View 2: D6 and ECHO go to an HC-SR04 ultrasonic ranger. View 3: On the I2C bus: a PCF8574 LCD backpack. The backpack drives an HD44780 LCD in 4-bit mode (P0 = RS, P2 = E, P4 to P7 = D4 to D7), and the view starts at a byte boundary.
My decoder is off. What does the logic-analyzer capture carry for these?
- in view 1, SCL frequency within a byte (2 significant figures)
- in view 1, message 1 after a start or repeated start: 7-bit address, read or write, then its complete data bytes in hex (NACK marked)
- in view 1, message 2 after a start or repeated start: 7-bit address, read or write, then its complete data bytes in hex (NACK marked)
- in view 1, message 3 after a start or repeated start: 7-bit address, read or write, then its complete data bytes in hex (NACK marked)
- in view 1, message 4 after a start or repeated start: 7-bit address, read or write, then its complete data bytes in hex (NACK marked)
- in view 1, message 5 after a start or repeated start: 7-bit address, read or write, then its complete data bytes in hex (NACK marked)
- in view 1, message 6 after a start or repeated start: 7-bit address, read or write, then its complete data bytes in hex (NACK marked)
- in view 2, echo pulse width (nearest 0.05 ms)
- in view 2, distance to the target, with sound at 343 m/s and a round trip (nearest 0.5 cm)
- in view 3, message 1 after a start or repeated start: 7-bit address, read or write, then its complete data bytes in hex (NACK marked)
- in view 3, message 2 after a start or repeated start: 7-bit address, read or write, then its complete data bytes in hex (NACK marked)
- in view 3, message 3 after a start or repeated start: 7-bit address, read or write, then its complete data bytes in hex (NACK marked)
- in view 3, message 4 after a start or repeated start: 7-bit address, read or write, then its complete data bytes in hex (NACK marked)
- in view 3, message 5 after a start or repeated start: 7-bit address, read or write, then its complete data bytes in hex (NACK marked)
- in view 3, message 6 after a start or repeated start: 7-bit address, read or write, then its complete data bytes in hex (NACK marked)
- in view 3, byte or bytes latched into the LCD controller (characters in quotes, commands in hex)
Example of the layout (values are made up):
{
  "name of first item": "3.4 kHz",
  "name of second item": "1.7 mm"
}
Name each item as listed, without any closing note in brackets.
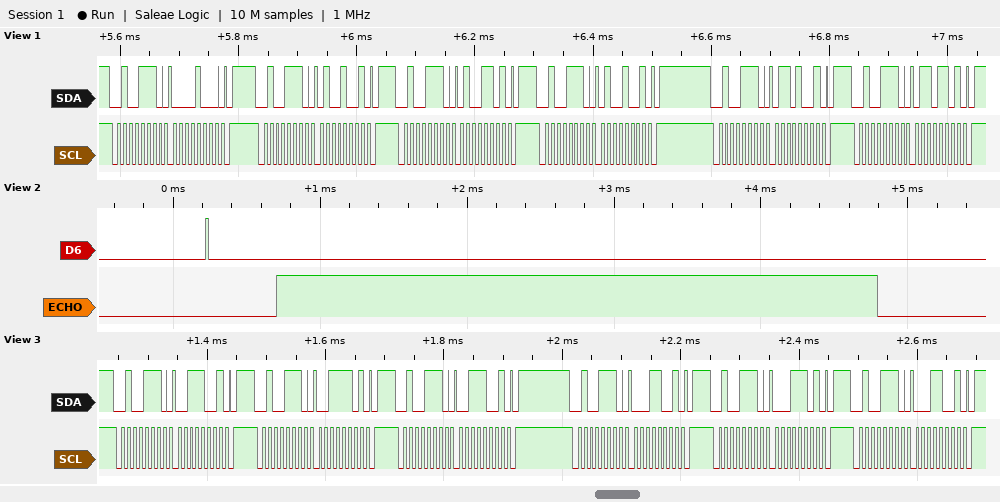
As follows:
{
  "in view 1, SCL frequency within a byte": "100 kHz",
  "in view 1, message 1 after a start or repeated start: 7-bit address, read or write, then its complete data bytes in hex": "0x27 write: 08",
  "in view 1, message 2 after a start or repeated start: 7-bit address, read or write, then its complete data bytes in hex": "0x27 write: 49",
  "in view 1, message 3 after a start or repeated start: 7-bit address, read or write, then its complete data bytes in hex": "0x27 write: 4D",
  "in view 1, message 4 after a start or repeated start: 7-bit address, read or write, then its complete data bytes in hex": "0x27 write: 49",
  "in view 1, message 5 after a start or repeated start: 7-bit address, read or write, then its complete data bytes in hex": "0x27 write: 69",
  "in view 1, message 6 after a start or repeated start: 7-bit address, read or write, then its complete data bytes in hex": "0x27 write: 6D",
  "in view 2, echo pulse width": "4.10 ms",
  "in view 2, distance to the target, with sound at 343 m/s and a round trip": "70 cm",
  "in view 3, message 1 after a start or repeated start: 7-bit address, read or write, then its complete data bytes in hex": "0x27 write: 39",
  "in view 3, message 2 after a start or repeated start: 7-bit address, read or write, then its complete data bytes in hex": "0x27 write: 3D",
  "in view 3, message 3 after a start or repeated start: 7-bit address, read or write, then its complete data bytes in hex": "0x27 write: 39",
  "in view 3, message 4 after a start or repeated start: 7-bit address, read or write, then its complete data bytes in hex": "0x27 write: 19",
  "in view 3, message 5 after a start or repeated start: 7-bit address, read or write, then its complete data bytes in hex": "0x27 write: 1D",
  "in view 3, message 6 after a start or repeated start: 7-bit address, read or write, then its complete data bytes in hex": "0x27 write: 19",
  "in view 3, byte or bytes latched into the LCD controller": "'1'"
}
